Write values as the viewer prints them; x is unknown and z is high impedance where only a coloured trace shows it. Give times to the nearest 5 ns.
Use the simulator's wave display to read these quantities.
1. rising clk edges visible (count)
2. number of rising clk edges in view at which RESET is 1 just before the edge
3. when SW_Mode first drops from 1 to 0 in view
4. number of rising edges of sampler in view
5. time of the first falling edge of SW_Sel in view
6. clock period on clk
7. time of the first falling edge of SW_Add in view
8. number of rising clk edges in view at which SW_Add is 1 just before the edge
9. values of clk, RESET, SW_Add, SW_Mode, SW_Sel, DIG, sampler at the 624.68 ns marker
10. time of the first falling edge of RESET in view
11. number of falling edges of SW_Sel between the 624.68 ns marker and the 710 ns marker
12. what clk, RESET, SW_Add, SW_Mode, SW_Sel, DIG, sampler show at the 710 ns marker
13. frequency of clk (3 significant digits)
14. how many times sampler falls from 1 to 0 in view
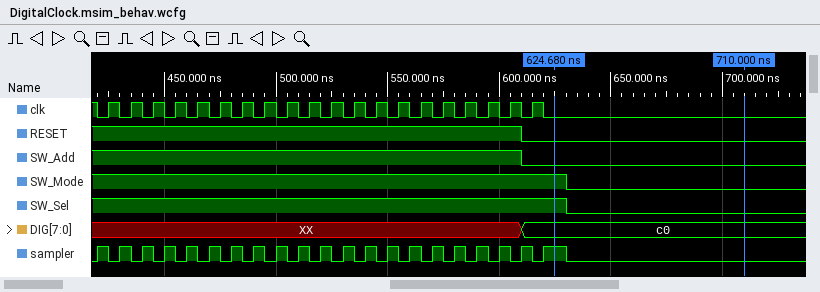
20
19
630 ns
21
630 ns
10 ns
610 ns
19
clk=0, RESET=0, SW_Add=0, SW_Mode=1, SW_Sel=1, DIG=c0, sampler=1
610 ns
1
clk=0, RESET=0, SW_Add=0, SW_Mode=0, SW_Sel=0, DIG=c0, sampler=0
100 MHz
21
